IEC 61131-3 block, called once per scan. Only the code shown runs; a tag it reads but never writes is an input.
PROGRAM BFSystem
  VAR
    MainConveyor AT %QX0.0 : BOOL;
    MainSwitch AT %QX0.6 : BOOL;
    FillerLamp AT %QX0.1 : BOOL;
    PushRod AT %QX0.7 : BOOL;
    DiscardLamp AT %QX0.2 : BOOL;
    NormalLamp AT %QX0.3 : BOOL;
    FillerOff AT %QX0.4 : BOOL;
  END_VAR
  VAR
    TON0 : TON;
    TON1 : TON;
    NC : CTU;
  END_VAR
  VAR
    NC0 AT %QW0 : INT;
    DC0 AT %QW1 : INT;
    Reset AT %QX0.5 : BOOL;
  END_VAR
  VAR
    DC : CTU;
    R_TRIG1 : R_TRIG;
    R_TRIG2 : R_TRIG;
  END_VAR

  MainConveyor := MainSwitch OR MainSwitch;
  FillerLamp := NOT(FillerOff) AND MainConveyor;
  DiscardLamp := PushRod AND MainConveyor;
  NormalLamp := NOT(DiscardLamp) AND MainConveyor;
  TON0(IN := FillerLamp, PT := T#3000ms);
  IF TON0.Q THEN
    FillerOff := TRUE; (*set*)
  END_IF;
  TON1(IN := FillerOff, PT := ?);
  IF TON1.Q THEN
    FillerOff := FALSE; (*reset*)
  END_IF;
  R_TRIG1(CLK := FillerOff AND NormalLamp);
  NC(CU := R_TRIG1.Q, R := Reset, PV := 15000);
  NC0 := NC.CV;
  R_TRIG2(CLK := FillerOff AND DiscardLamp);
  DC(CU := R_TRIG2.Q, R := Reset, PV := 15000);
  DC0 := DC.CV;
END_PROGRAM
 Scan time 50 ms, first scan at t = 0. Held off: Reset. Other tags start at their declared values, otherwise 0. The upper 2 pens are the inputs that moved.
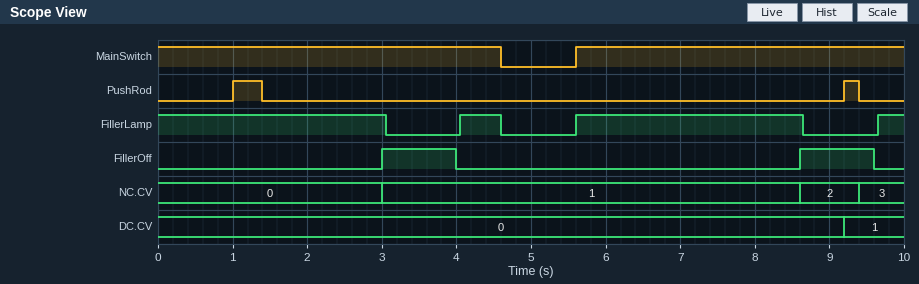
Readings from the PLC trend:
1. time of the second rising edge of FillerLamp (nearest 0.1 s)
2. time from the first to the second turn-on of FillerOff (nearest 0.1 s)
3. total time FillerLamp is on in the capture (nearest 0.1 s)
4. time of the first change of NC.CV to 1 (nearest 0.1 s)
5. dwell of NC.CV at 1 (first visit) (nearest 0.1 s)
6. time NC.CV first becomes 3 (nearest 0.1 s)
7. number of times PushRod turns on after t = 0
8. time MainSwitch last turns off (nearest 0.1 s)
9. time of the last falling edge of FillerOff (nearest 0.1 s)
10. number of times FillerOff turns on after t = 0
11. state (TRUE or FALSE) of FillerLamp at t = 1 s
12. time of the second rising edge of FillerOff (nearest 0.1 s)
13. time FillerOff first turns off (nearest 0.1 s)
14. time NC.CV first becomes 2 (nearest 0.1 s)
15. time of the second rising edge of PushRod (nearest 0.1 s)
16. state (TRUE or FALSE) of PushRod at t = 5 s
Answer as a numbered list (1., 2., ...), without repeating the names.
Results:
1. 5.6 s
2. 5.6 s
3. 7.0 s
4. 3.0 s
5. 5.6 s
6. 9.4 s
7. 2
8. 4.6 s
9. 9.6 s
10. 2
11. TRUE
12. 8.6 s
13. 4.0 s
14. 8.6 s
15. 9.2 s
16. FALSE
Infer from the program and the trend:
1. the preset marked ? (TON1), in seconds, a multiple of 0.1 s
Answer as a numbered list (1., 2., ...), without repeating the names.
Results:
1. 1.0 s
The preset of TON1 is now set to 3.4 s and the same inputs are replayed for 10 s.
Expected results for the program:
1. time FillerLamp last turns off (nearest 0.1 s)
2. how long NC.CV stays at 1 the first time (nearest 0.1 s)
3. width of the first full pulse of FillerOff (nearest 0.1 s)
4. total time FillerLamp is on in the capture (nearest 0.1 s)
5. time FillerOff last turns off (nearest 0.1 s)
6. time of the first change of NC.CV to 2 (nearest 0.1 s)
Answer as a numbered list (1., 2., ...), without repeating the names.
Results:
1. 9.5 s
2. 2.6 s
3. 3.4 s
4. 6.1 s
5. 6.4 s
6. 5.6 s
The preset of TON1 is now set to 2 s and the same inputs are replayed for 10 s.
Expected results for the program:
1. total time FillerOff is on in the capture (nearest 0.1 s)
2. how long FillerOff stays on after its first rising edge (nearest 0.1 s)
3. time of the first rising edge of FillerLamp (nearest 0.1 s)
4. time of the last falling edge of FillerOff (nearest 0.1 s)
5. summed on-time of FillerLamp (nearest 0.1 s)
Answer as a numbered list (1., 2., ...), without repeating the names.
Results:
1. 3.4 s
2. 2.0 s
3. 5.6 s
4. 5.0 s
5. 6.1 s
